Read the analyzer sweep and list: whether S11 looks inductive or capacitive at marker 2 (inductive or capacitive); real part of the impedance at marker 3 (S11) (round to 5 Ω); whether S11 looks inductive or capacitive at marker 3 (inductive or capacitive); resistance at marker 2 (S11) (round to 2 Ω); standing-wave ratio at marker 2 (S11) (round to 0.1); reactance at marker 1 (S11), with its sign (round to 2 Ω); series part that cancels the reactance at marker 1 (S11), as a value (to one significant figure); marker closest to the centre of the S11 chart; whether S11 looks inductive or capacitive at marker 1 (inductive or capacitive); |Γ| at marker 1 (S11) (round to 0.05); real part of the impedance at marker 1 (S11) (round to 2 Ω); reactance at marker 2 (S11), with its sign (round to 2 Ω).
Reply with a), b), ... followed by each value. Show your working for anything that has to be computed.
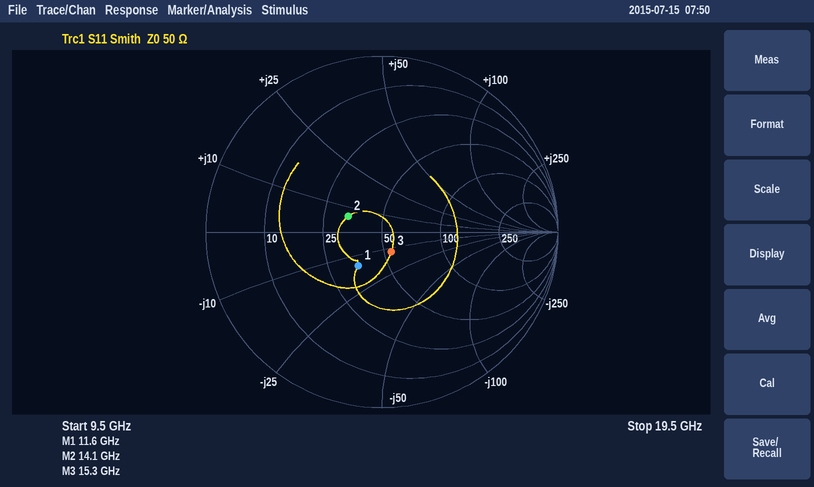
a) inductive
b) 55 Ω
c) capacitive
d) 34 Ω
e) 1.5
f) -14 Ω
g) L = 14 Ω/(2π × 11.6 GHz) ≈ 192 pH, so 200 pH to one significant figure
h) marker 3
i) capacitive
j) 0.25
k) 36 Ω
l) +6 Ω
